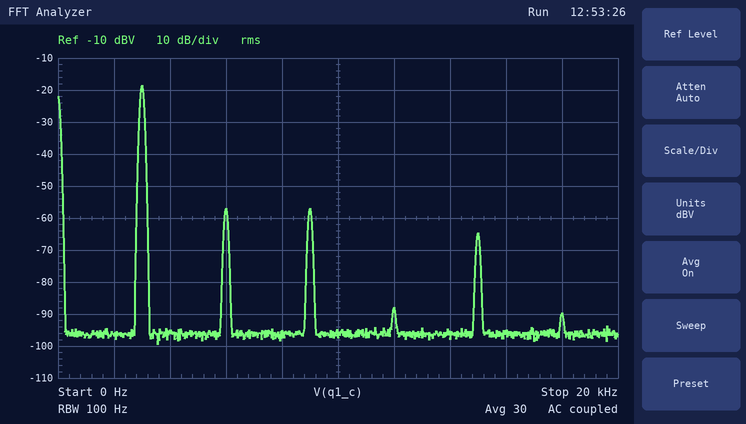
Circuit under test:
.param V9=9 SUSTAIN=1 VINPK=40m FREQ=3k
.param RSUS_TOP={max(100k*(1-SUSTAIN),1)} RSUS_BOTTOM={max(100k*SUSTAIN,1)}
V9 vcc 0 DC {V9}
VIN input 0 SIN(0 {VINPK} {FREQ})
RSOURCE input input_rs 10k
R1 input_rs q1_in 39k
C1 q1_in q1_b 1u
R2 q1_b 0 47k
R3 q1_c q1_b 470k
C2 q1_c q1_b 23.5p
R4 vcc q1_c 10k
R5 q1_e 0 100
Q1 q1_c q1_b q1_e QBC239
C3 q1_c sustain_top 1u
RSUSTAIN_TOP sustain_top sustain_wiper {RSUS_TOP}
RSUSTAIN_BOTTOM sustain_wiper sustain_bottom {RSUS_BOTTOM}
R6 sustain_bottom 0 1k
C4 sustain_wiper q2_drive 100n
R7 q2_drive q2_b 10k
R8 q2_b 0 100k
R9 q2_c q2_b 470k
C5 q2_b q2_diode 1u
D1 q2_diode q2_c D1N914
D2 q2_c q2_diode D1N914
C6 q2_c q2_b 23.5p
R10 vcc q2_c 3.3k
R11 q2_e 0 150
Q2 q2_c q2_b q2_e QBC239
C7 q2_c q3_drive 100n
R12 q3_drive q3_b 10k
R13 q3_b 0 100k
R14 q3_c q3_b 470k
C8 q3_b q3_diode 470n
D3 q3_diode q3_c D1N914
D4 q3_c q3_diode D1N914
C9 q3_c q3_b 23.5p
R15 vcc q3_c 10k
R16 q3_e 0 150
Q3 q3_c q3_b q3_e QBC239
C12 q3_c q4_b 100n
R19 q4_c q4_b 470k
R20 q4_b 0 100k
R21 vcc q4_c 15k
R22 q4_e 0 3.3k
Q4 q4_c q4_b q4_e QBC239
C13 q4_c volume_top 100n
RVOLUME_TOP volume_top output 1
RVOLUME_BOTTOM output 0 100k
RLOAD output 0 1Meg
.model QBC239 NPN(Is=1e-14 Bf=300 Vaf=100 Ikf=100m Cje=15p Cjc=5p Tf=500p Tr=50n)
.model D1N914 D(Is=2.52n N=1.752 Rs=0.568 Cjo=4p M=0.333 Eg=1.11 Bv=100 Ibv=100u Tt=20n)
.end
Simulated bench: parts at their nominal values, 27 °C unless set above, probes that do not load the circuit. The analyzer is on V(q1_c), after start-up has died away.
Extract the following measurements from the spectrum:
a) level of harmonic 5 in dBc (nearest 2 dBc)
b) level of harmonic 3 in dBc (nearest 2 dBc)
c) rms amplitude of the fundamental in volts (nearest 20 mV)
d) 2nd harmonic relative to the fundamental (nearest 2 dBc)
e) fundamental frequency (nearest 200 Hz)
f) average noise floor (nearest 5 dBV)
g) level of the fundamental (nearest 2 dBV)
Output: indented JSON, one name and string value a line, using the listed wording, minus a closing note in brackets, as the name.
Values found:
{
  "level of harmonic 5 in dBc": "-46 dBc",
  "level of harmonic 3 in dBc": "-38 dBc",
  "rms amplitude of the fundamental in volts": "120 mV",
  "2nd harmonic relative to the fundamental": "-38 dBc",
  "fundamental frequency": "3.0 kHz",
  "average noise floor": "-95 dBV",
  "level of the fundamental": "-18 dBV"
}
